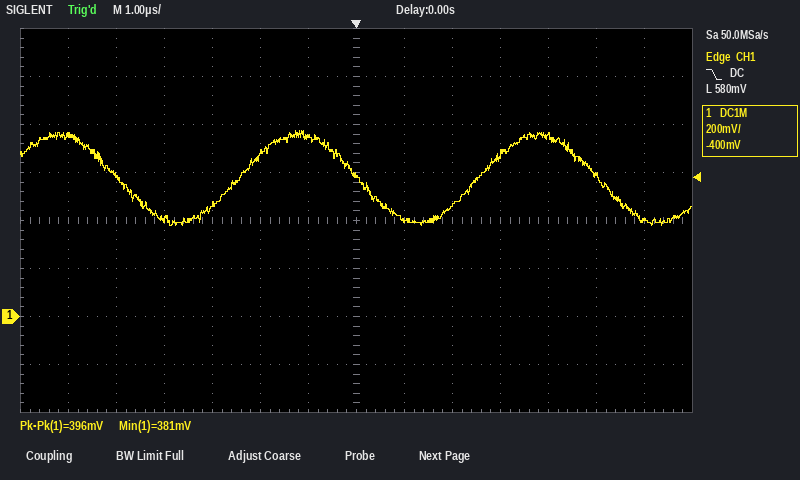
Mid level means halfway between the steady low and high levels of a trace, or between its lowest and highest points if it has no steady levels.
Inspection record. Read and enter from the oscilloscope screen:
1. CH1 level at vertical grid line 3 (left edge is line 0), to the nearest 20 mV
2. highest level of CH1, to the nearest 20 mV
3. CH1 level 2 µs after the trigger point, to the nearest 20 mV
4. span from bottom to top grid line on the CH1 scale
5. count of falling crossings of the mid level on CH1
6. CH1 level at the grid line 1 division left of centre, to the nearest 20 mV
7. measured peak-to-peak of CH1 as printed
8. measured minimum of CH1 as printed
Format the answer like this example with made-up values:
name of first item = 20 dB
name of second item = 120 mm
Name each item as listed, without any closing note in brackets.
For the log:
CH1 level at vertical grid line 3 (left edge is line 0), to the nearest 20 mV = 400 mV
highest level of CH1, to the nearest 20 mV = 780 mV
CH1 level 2 µs after the trigger point, to the nearest 20 mV = 460 mV
span from bottom to top grid line on the CH1 scale = 1.6 V
count of falling crossings of the mid level on CH1 = 3
CH1 level at the grid line 1 division left of centre, to the nearest 20 mV = 740 mV
measured peak-to-peak of CH1 as printed = 396 mV
measured minimum of CH1 as printed = 381 mV
